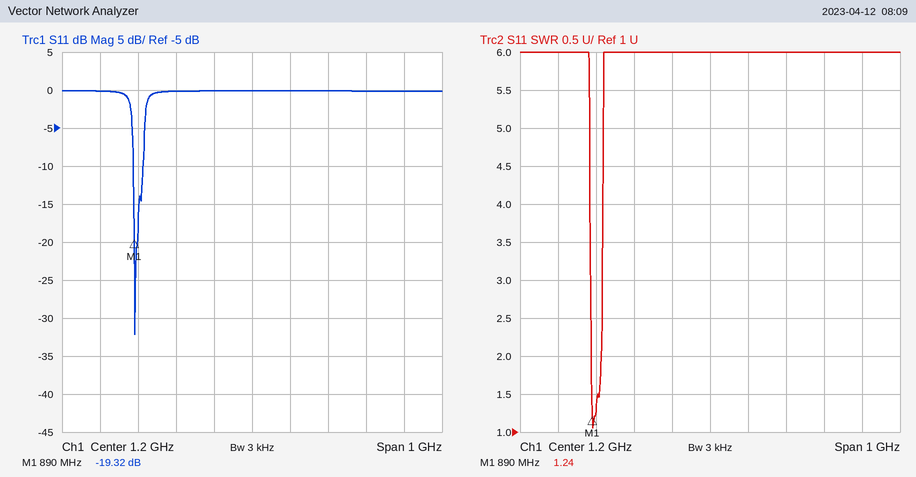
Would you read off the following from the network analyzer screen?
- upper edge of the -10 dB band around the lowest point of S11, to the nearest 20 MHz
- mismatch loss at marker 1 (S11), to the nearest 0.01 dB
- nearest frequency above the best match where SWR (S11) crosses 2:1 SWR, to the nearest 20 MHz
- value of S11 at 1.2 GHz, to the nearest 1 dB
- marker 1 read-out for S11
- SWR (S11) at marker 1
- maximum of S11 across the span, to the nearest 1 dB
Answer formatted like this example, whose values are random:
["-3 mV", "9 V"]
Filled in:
["920 MHz", "0.05 dB", "920 MHz", "0 dB", "-19.32 dB", "1.24", "0 dB"]
